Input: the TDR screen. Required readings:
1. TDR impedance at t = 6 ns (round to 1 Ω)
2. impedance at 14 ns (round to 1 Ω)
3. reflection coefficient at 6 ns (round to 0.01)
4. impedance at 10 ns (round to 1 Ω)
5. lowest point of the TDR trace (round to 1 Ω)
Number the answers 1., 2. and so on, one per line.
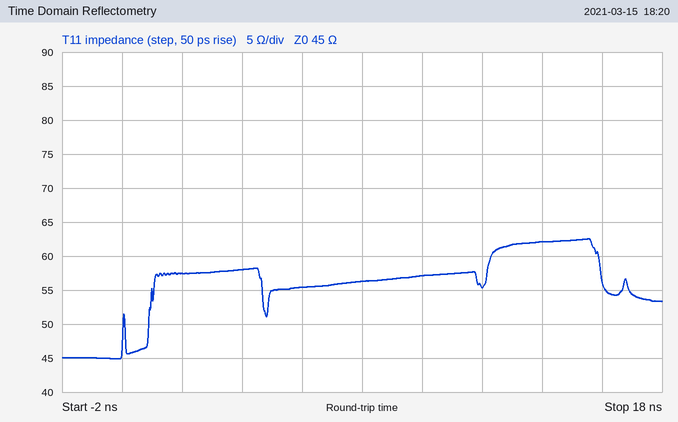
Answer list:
1. 55 Ω
2. 62 Ω
3. +0.10
4. 57 Ω
5. 45 Ω
